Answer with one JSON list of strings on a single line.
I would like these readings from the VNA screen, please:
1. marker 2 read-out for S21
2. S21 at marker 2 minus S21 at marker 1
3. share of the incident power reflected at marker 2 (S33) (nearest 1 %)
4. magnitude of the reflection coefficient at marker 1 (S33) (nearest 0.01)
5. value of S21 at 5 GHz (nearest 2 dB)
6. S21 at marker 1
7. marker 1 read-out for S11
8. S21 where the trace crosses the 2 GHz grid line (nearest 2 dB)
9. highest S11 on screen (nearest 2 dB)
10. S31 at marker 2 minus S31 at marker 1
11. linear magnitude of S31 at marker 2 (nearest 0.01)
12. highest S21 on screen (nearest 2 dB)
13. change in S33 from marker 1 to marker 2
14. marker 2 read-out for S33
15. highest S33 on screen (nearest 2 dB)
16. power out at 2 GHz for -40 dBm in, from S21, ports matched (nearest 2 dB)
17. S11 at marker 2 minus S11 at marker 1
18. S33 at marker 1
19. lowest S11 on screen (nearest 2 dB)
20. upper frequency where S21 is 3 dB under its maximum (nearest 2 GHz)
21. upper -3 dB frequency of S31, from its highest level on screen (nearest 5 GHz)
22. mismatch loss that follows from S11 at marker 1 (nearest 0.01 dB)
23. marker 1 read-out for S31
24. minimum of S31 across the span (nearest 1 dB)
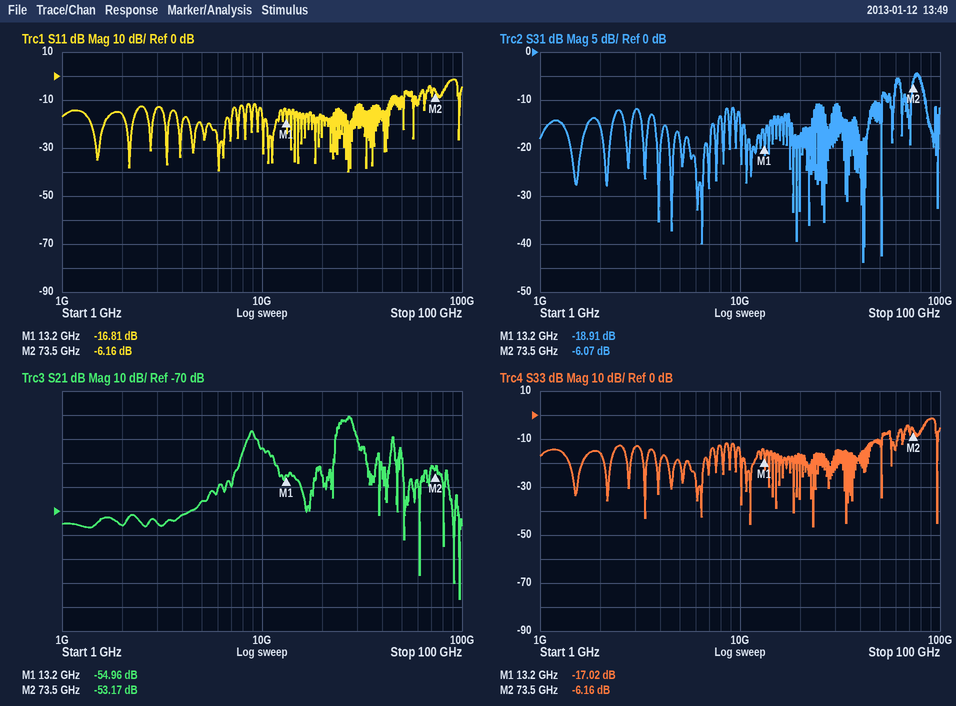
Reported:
["-53.17 dB", "1.79 dB", "24 %", "0.14", "-66 dB", "-54.96 dB", "-16.81 dB", "-76 dB", "-2 dB", "12.84 dB", "0.50", "-30 dB", "10.86 dB", "-6.16 dB", "-2 dB", "-116 dBm", "10.65 dB", "-17.02 dB", "-40 dB", "28 GHz", "80 GHz", "0.09 dB", "-18.91 dB", "-44 dB"]
